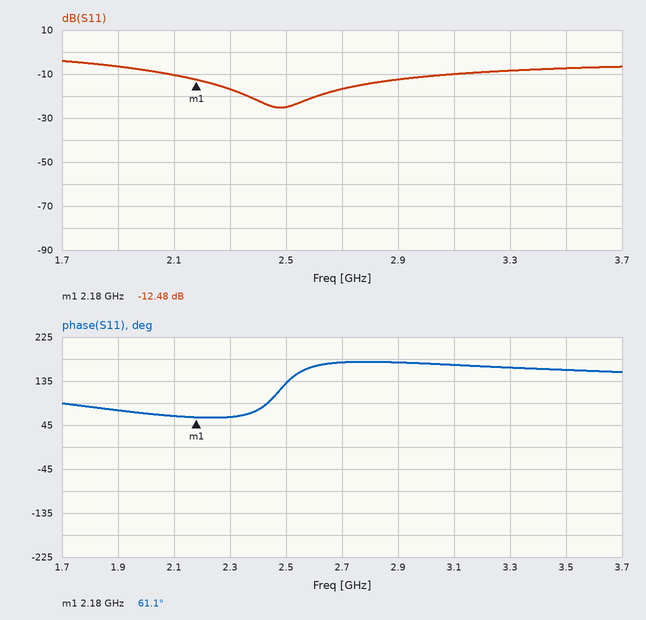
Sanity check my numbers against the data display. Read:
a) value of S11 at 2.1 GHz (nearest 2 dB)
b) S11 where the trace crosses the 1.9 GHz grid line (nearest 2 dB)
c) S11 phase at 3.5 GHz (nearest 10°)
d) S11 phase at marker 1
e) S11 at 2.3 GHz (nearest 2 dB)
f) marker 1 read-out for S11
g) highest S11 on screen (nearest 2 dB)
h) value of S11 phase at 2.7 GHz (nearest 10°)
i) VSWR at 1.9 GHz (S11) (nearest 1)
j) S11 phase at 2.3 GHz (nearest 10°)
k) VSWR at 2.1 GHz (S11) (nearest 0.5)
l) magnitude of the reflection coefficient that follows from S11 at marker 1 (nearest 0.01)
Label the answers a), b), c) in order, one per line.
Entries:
a) -10 dB
b) -6 dB
c) 160°
d) 61.1°
e) -16 dB
f) -12.48 dB
g) -4 dB
h) 170°
i) 3
j) 60°
k) 2.0
l) 0.24
